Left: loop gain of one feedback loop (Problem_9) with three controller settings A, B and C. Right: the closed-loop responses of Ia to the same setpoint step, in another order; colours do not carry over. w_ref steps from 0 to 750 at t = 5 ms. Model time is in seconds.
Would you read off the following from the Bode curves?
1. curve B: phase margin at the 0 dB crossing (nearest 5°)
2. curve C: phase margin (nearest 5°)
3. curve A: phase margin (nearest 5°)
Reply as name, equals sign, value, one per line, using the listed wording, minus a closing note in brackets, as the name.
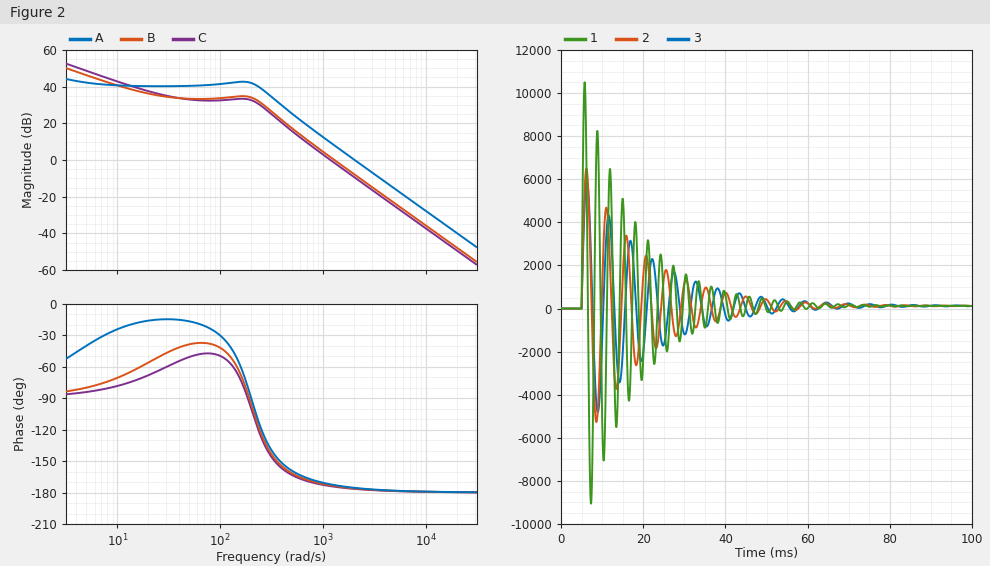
curve B: phase margin at the 0 dB crossing = 5°
curve C: phase margin = 5°
curve A: phase margin = 5°
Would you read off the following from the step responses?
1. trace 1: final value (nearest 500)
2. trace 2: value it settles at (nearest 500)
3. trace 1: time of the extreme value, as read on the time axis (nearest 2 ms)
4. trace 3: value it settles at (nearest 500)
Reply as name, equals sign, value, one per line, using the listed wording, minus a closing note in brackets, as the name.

trace 1: final value = 0
trace 2: value it settles at = 0
trace 1: time of the extreme value, as read on the time axis = 6 ms
trace 3: value it settles at = 0
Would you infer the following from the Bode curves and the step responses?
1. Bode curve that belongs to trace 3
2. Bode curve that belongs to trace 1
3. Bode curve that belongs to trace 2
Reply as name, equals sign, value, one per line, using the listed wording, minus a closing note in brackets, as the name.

Bode curve that belongs to trace 3 = C
Bode curve that belongs to trace 1 = A
Bode curve that belongs to trace 2 = B
